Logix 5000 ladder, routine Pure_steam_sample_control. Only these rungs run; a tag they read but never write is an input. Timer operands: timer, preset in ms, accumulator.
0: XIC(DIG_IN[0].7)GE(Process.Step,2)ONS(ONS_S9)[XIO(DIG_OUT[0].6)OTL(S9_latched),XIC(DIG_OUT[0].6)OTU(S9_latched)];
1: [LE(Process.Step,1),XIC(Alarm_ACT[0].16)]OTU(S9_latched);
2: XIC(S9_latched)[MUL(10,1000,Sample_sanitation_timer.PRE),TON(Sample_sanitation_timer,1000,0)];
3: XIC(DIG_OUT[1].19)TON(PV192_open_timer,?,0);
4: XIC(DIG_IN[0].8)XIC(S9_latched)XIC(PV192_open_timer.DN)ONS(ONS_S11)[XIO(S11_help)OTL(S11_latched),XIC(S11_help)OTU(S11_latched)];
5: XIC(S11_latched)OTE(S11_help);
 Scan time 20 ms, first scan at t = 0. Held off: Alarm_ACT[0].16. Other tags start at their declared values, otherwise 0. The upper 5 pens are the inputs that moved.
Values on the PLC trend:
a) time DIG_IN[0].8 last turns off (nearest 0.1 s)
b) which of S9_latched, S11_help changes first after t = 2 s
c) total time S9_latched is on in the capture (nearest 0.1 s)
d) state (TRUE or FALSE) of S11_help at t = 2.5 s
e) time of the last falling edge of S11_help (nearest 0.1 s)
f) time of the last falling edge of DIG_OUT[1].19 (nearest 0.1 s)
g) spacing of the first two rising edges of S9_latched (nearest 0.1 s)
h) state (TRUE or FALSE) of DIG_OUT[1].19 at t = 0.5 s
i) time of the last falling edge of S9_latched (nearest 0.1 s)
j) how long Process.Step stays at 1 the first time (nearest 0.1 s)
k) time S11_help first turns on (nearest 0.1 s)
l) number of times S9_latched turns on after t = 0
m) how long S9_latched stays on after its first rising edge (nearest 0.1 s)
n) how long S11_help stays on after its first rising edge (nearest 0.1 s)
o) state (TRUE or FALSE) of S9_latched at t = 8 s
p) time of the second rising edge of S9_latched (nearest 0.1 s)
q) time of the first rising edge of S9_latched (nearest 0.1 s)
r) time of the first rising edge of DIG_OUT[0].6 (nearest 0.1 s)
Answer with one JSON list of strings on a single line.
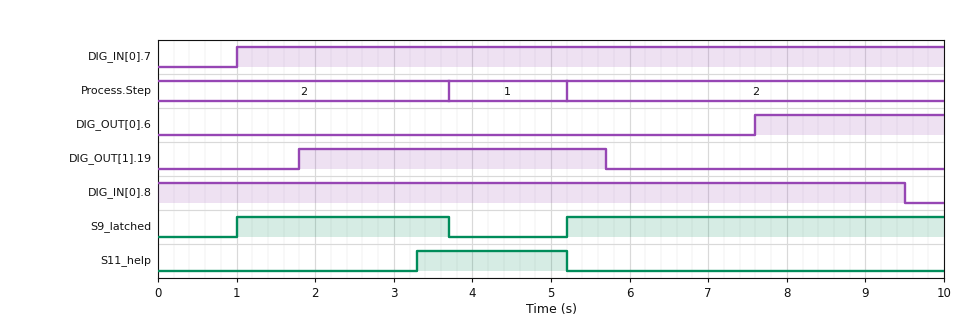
["9.5 s", "S11_help", "7.5 s", "FALSE", "5.2 s", "5.7 s", "4.2 s", "FALSE", "3.7 s", "1.5 s", "3.3 s", "2", "2.7 s", "1.9 s", "TRUE", "5.2 s", "1.0 s", "7.6 s"]
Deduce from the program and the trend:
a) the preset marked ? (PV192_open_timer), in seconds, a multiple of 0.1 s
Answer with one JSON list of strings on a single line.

["1.5 s"]
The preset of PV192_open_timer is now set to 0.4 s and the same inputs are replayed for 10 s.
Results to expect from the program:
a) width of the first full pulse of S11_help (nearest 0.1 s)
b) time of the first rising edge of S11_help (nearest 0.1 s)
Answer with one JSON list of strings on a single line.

["3.0 s", "2.2 s"]
